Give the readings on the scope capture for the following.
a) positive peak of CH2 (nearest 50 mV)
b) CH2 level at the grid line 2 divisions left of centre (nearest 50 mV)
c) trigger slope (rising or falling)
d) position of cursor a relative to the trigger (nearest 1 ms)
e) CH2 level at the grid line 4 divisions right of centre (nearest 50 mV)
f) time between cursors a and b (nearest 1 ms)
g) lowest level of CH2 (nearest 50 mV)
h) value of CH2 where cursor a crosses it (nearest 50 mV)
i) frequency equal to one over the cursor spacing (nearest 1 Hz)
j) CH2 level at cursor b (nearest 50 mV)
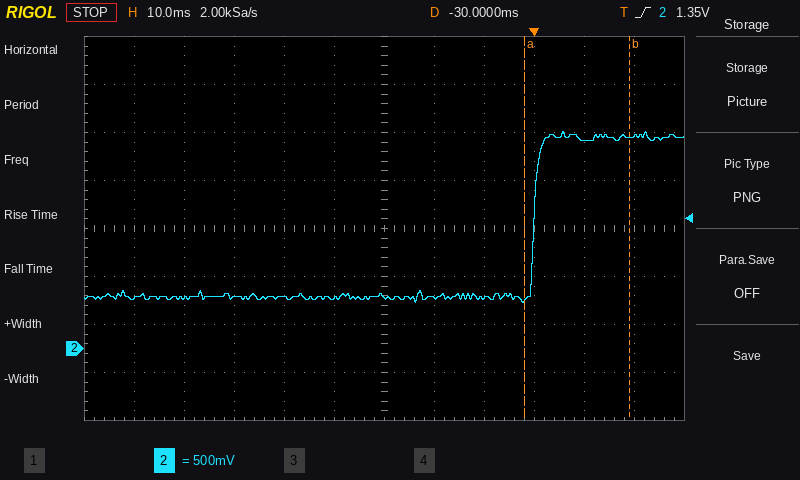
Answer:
2.25 V
550 mV
rising
-2 ms
2.15 V
21 ms
500 mV
500 mV
48 Hz
2.20 V
